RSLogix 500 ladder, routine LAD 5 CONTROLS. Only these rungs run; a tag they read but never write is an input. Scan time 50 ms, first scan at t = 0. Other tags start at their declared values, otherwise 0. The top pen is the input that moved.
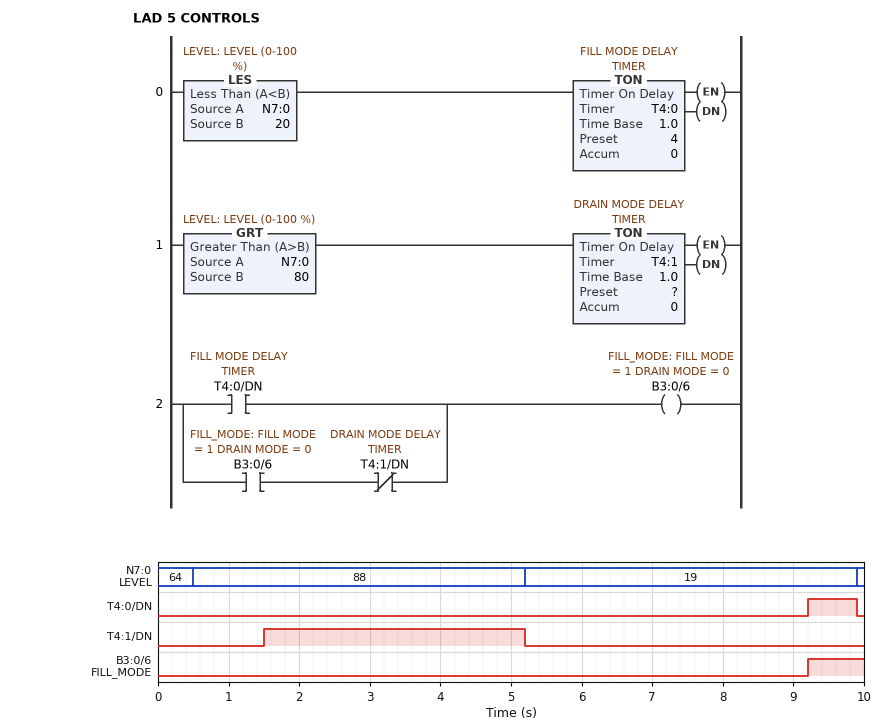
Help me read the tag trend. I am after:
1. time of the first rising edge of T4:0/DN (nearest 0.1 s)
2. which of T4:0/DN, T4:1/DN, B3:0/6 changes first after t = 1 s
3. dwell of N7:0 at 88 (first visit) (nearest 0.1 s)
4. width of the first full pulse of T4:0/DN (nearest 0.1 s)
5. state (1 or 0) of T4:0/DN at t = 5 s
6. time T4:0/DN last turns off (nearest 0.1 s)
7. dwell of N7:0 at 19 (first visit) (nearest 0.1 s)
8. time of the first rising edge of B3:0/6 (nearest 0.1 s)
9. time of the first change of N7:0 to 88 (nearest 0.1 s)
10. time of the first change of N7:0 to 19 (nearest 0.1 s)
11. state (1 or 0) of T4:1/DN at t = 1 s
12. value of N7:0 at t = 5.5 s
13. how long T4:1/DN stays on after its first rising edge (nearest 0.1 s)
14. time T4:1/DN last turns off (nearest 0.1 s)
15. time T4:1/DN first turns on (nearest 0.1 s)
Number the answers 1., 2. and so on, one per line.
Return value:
1. 9.2 s
2. T4:1/DN
3. 4.7 s
4. 0.7 s
5. 0
6. 9.9 s
7. 4.7 s
8. 9.2 s
9. 0.5 s
10. 5.2 s
11. 0
12. 19
13. 3.7 s
14. 5.2 s
15. 1.5 s
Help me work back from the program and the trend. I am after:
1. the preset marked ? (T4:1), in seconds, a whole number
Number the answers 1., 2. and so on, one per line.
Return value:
1. 1 s
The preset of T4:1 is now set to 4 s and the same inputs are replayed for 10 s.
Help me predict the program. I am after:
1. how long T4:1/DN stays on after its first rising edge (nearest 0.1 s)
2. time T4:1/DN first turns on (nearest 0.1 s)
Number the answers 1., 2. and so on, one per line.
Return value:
1. 0.7 s
2. 4.5 s
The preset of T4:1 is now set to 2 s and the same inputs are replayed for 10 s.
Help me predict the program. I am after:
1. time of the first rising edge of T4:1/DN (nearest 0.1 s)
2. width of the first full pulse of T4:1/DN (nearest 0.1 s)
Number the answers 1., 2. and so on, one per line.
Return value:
1. 2.5 s
2. 2.7 s
